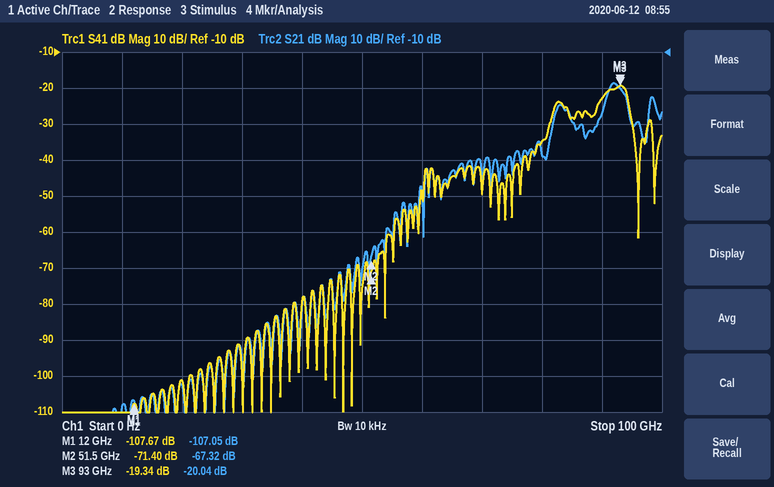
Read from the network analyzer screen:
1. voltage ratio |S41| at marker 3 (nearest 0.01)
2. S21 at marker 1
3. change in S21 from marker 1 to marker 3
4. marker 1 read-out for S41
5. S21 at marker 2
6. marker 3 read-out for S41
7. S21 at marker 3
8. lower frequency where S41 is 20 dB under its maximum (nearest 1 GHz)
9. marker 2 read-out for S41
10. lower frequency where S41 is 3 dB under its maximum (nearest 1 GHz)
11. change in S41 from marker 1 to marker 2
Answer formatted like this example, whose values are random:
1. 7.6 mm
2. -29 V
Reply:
1. 0.11
2. -107.05 dB
3. 87.01 dB
4. -107.67 dB
5. -67.32 dB
6. -19.34 dB
7. -20.04 dB
8. 78 GHz
9. -71.40 dB
10. 90 GHz
11. 36.27 dB
